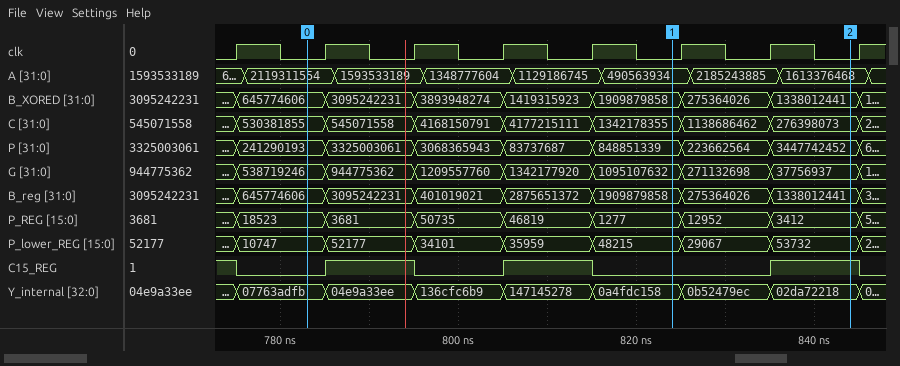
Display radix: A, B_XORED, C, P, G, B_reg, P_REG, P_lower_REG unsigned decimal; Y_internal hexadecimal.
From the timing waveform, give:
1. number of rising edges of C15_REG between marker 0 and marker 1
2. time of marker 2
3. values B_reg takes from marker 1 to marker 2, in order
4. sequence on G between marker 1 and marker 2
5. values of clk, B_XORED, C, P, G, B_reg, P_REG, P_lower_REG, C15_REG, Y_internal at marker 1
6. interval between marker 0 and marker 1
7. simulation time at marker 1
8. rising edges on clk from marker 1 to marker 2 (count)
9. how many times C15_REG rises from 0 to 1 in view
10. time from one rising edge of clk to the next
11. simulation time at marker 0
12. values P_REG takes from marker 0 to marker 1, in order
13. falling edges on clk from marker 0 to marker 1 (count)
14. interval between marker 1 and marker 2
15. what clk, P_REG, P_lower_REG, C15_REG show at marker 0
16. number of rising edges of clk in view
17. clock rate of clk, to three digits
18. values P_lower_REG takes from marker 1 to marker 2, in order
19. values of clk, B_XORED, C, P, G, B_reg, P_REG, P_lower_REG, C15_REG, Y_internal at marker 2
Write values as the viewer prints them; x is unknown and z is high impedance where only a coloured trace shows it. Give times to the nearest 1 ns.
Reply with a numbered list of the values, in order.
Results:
1. 2
2. 844 ns
3. 1909879858, 275364026, 1338012441
4. 1095107632, 271132698, 37756937
5. clk=0, B_XORED=1909879858, C=1342178355, P=848851339, G=1095107632, B_reg=1909879858, P_REG=1277, P_lower_REG=48215, C15_REG=0, Y_internal=0a4fdc158
6. 41 ns
7. 824 ns
8. 2
9. 3
10. 10 ns
11. 783 ns
12. 18523, 3681, 50735, 46819, 1277
13. 4
14. 20 ns
15. clk=0, P_REG=18523, P_lower_REG=10747, C15_REG=0
16. 8
17. 100 MHz
18. 48215, 29067, 53732
19. clk=0, B_XORED=1338012441, C=276398073, P=3447742452, G=37756937, B_reg=1338012441, P_REG=3412, P_lower_REG=53732, C15_REG=1, Y_internal=02da72218
